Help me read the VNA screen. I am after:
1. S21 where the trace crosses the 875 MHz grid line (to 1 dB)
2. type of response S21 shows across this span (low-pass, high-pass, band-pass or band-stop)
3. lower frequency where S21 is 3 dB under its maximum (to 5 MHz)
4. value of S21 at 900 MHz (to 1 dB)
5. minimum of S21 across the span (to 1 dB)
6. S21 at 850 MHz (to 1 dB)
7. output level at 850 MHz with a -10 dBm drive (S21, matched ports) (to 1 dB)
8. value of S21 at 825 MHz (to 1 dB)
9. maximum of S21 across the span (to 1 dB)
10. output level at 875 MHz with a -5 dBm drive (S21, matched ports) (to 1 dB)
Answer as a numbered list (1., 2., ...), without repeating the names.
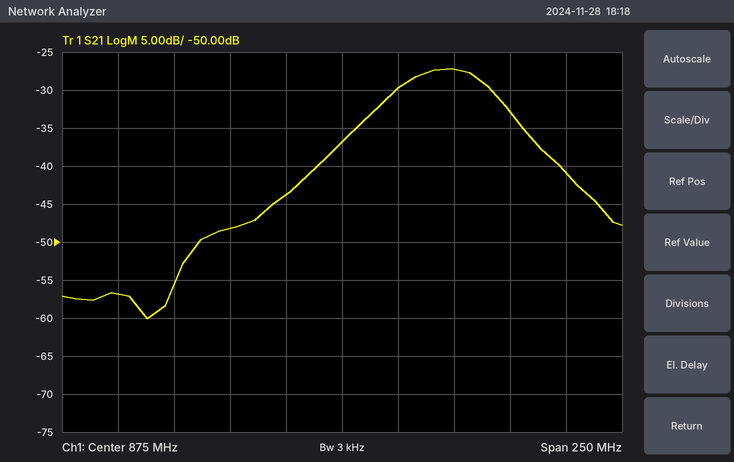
1. -37 dB
2. band-pass
3. 900 MHz
4. -30 dB
5. -60 dB
6. -44 dB
7. -54 dBm
8. -48 dB
9. -27 dB
10. -42 dBm
